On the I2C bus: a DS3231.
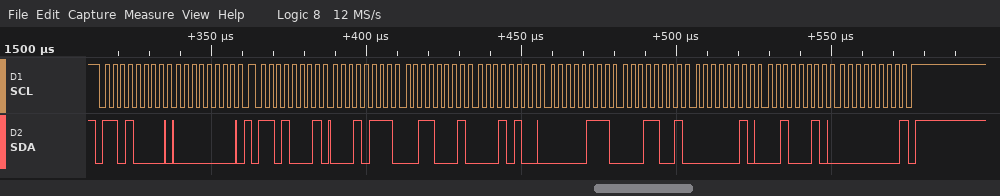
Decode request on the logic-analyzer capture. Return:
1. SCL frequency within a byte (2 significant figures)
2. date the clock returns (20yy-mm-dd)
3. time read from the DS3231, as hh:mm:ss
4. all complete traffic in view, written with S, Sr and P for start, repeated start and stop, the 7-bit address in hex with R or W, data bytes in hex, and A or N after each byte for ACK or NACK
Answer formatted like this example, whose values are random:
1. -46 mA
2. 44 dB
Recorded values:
1. 400 kHz
2. 2022-02-19
3. 14:31:17
4. S 68W A 00 A Sr 68R A 17 A 31 A 14 A 07 A 19 A 02 A 22 A 00 N P
